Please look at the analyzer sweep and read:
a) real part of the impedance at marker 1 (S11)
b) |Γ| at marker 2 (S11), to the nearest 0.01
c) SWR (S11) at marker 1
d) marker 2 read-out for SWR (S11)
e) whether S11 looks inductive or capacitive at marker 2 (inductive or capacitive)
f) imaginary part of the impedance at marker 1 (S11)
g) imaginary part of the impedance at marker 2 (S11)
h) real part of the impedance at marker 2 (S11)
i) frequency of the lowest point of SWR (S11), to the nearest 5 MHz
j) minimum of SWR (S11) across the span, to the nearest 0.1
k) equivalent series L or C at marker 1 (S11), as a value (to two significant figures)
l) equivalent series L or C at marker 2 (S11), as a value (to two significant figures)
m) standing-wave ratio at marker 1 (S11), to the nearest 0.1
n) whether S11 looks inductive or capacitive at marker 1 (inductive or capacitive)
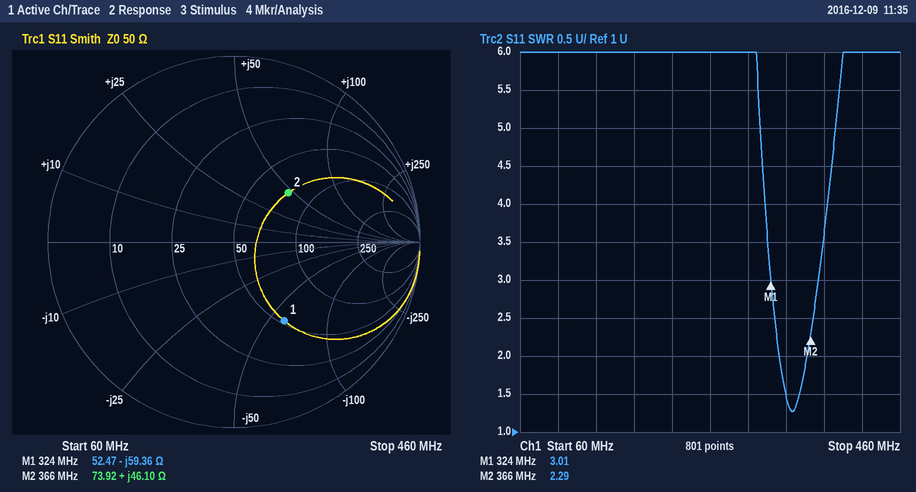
52.47 Ω
0.39
3.01
2.29
inductive
-59.36 Ω
+46.10 Ω
73.92 Ω
345 MHz
1.3
8.3 pF
20 nH
3.0
capacitive
